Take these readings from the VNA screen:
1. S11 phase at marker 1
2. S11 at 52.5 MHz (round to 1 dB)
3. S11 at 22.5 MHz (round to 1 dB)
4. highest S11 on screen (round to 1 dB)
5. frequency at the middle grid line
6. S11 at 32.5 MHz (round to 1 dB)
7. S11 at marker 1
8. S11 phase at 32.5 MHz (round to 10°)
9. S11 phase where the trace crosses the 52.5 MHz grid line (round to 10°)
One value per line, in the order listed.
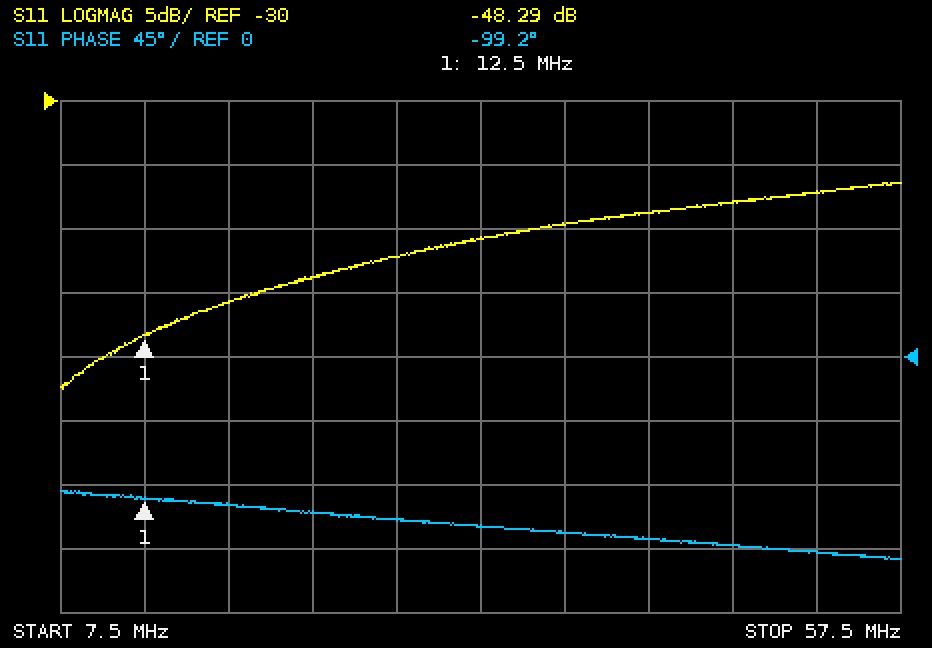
-99.2°
-37 dB
-44 dB
-36 dB
32.5 MHz
-41 dB
-48.29 dB
-120°
-140°
